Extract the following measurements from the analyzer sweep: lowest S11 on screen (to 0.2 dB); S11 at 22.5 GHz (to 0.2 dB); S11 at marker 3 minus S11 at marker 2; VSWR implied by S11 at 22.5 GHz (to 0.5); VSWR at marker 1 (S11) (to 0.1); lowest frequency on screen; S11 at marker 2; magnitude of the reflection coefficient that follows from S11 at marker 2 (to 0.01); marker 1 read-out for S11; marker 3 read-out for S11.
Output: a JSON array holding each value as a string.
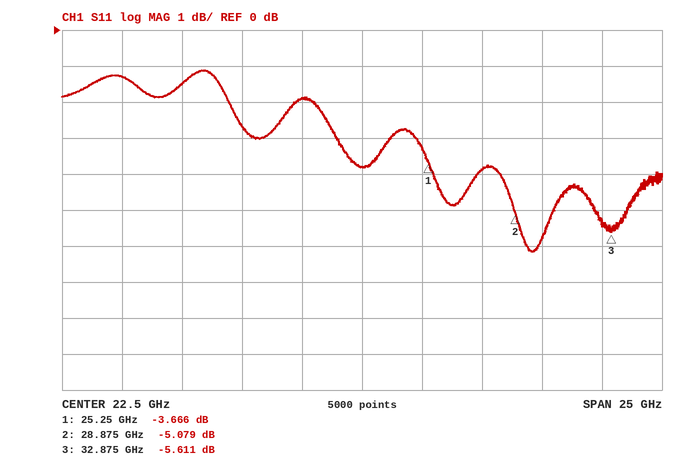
["-6.2 dB", "-3.8 dB", "-0.532 dB", "4.5", "4.8", "10 GHz", "-5.079 dB", "0.56", "-3.666 dB", "-5.611 dB"]
